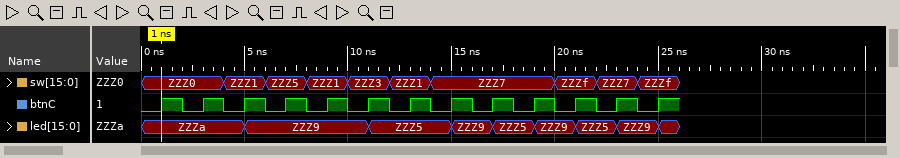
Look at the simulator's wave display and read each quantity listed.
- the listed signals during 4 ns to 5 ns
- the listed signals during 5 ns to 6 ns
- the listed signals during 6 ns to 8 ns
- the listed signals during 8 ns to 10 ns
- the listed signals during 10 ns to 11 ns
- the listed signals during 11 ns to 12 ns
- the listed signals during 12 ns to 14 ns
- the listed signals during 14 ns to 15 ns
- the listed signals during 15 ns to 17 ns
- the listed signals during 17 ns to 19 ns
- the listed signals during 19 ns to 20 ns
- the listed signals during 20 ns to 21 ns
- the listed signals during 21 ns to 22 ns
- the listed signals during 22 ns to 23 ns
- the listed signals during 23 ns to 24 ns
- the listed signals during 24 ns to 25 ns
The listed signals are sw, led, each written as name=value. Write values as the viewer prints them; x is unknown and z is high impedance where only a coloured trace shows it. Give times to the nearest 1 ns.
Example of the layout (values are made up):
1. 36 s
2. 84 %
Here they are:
1. sw=ZZZ1, led=ZZZa
2. sw=ZZZ1, led=ZZZ9
3. sw=ZZZ5, led=ZZZ9
4. sw=ZZZ1, led=ZZZ9
5. sw=ZZZ3, led=ZZZ9
6. sw=ZZZ3, led=ZZZ5
7. sw=ZZZ1, led=ZZZ5
8. sw=ZZZ7, led=ZZZ5
9. sw=ZZZ7, led=ZZZ9
10. sw=ZZZ7, led=ZZZ5
11. sw=ZZZ7, led=ZZZ9
12. sw=ZZZf, led=ZZZ9
13. sw=ZZZf, led=ZZZ5
14. sw=ZZZ7, led=ZZZ5
15. sw=ZZZ7, led=ZZZ9
16. sw=ZZZf, led=ZZZ9
